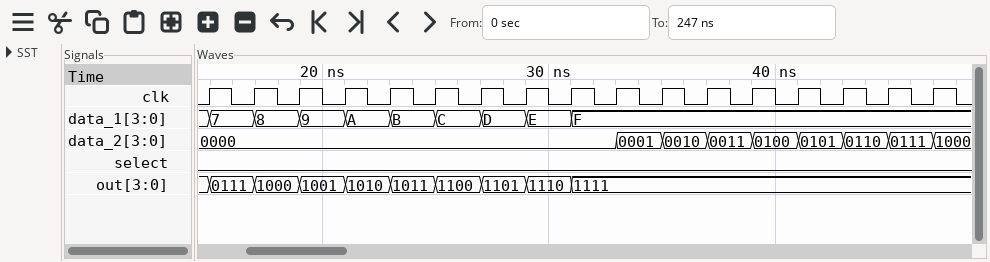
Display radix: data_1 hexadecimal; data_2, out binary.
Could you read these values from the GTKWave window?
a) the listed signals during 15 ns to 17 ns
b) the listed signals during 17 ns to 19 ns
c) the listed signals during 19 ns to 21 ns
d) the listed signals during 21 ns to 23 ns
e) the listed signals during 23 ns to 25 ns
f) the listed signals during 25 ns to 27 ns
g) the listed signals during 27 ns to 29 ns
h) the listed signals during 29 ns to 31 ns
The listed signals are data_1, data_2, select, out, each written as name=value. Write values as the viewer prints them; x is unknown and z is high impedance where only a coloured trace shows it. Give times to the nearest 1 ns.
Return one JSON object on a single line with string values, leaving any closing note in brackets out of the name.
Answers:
{"the listed signals during 15 ns to 17 ns": "data_1=7, data_2=0000, select=0, out=0111", "the listed signals during 17 ns to 19 ns": "data_1=8, data_2=0000, select=0, out=1000", "the listed signals during 19 ns to 21 ns": "data_1=9, data_2=0000, select=0, out=1001", "the listed signals during 21 ns to 23 ns": "data_1=A, data_2=0000, select=0, out=1010", "the listed signals during 23 ns to 25 ns": "data_1=B, data_2=0000, select=0, out=1011", "the listed signals during 25 ns to 27 ns": "data_1=C, data_2=0000, select=0, out=1100", "the listed signals during 27 ns to 29 ns": "data_1=D, data_2=0000, select=0, out=1101", "the listed signals during 29 ns to 31 ns": "data_1=E, data_2=0000, select=0, out=1110"}
